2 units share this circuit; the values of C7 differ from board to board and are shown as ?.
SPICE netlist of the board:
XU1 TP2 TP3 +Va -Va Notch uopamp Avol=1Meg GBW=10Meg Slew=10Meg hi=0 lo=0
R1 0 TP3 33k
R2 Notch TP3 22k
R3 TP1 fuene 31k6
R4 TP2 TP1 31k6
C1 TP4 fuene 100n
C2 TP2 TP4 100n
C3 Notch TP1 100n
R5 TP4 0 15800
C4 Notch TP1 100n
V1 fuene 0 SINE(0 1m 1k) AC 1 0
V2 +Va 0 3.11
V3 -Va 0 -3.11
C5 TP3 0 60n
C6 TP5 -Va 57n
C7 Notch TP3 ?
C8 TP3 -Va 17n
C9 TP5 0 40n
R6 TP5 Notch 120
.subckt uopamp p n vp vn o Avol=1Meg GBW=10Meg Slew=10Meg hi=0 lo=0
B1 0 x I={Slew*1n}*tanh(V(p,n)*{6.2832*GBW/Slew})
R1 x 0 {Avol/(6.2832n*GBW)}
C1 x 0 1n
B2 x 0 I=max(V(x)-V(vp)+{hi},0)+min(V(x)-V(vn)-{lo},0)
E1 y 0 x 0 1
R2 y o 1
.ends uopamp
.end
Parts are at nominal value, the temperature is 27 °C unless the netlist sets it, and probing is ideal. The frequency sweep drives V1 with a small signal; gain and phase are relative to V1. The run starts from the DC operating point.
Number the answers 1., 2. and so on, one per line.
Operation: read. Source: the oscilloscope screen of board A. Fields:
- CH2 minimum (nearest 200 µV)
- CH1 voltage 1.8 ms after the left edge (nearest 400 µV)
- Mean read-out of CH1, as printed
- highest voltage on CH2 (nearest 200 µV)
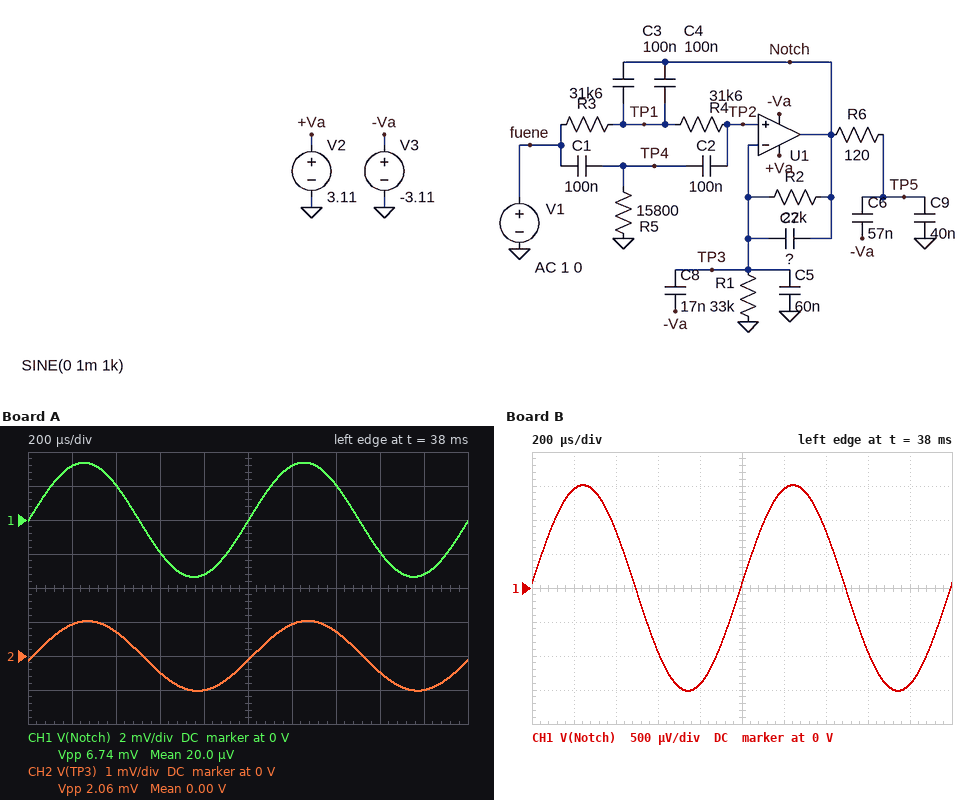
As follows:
1. -1.0 mV
2. -3.2 mV
3. 20.0 µV
4. 1.0 mV
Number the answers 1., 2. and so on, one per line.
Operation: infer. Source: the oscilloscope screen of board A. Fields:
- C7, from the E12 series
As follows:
1. 33 nF
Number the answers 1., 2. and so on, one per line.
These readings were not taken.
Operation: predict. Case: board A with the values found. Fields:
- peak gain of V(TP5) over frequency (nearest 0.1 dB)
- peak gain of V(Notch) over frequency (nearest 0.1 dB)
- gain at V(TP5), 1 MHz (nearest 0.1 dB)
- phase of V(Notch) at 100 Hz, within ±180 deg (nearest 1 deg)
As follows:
1. 22.9 dB
2. 22.9 dB
3. -26.9 dB
4. 40 deg
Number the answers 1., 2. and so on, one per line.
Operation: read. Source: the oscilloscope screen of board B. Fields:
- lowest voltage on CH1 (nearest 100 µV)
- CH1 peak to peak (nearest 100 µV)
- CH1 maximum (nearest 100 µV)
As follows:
1. -1.5 mV
2. 3.0 mV
3. 1.5 mV
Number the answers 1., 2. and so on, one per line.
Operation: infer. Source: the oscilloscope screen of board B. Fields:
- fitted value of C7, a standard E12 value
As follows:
1. 150 nF
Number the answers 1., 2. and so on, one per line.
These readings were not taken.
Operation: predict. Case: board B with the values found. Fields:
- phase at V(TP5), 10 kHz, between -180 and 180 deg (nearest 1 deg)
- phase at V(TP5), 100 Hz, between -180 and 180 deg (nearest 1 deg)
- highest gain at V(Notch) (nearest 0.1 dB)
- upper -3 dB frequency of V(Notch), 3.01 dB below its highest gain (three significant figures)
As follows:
1. -36 deg
2. 27 deg
3. 7.3 dB
4. 5.40 MHz
